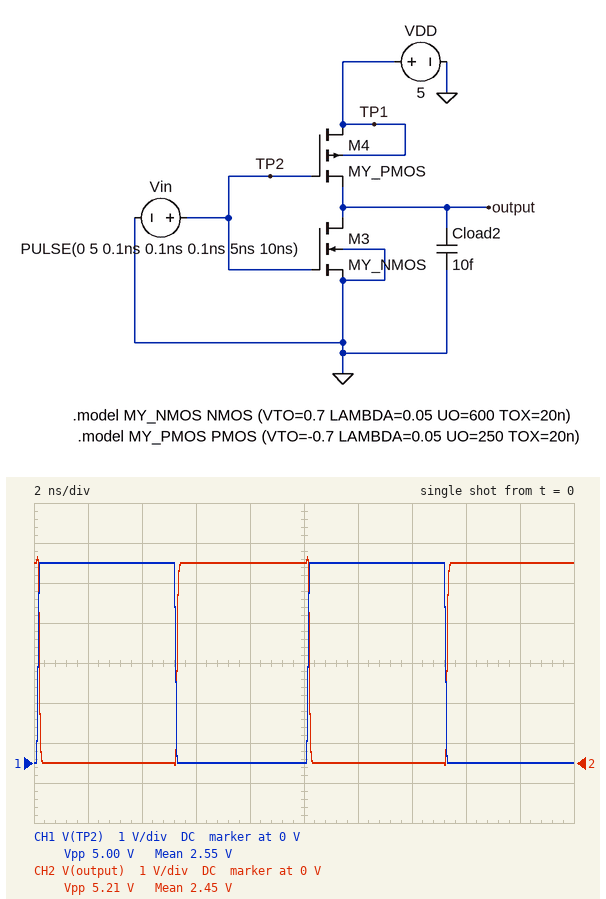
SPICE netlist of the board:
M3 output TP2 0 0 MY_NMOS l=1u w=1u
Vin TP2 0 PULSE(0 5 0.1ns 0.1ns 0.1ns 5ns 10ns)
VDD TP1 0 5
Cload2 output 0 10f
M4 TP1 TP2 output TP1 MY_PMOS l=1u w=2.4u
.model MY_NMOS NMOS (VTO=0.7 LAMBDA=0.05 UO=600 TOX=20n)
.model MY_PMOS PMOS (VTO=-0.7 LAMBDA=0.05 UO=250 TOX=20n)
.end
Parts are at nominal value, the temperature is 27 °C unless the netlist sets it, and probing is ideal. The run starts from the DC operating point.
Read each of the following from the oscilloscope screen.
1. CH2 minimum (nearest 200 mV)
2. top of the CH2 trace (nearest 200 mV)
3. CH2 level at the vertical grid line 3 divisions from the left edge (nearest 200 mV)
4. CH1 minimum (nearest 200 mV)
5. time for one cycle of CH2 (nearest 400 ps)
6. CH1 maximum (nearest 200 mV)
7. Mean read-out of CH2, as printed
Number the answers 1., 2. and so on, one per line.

1. 0 V
2. 5.2 V
3. 5.0 V
4. 0 V
5. 10.0 ns
6. 5.0 V
7. 2.45 V
